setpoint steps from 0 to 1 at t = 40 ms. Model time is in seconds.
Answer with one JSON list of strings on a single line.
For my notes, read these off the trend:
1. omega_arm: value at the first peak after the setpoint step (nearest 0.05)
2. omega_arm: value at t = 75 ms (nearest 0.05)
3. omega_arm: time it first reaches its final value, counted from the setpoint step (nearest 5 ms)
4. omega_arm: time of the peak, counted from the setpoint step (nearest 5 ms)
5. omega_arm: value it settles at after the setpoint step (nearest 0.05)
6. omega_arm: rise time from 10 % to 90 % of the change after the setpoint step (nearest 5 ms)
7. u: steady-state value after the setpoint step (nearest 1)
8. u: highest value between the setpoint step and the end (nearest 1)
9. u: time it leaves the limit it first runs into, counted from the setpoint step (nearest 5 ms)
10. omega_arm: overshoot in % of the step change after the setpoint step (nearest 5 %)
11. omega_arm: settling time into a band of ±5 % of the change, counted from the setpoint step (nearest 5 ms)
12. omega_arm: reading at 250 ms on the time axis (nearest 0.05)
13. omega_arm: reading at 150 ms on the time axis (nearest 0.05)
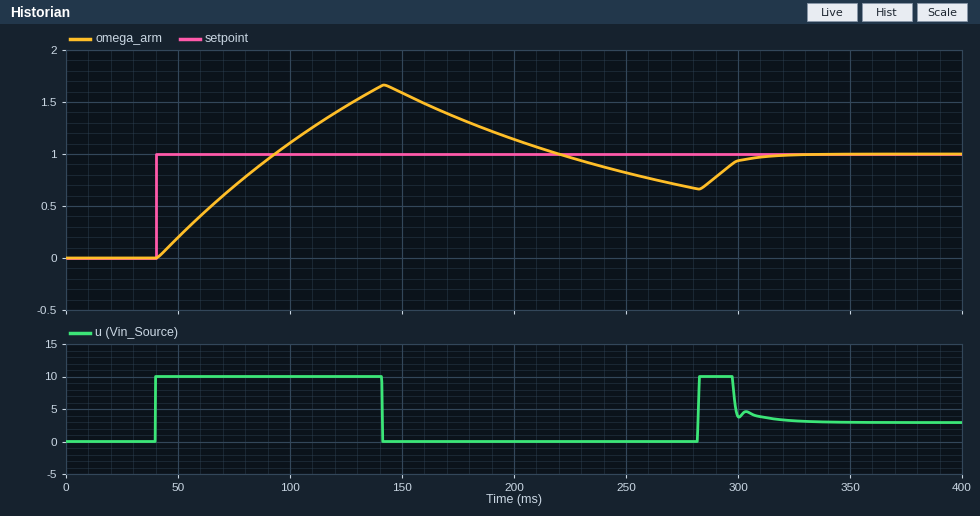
["1.65", "0.70", "55 ms", "100 ms", "1.00", "40 ms", "3", "10", "100 ms", "65 %", "265 ms", "0.80", "1.60"]
